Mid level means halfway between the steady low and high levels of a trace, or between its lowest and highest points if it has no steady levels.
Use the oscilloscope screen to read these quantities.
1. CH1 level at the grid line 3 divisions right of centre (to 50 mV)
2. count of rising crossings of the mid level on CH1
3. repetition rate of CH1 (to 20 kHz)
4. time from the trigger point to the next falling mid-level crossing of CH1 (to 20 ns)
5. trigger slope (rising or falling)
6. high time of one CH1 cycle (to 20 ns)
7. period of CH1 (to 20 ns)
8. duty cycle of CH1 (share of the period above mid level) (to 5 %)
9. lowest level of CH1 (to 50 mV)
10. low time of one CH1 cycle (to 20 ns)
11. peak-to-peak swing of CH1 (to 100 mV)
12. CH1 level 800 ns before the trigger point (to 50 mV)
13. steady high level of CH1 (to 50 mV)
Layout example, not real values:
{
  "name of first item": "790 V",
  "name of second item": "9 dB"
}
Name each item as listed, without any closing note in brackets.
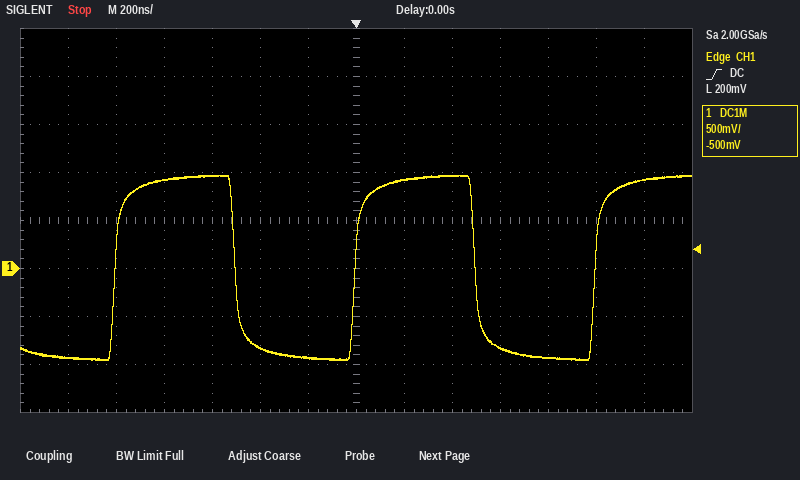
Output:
{
  "CH1 level at the grid line 3 divisions right of centre": "-850 mV",
  "count of rising crossings of the mid level on CH1": "3",
  "repetition rate of CH1": "1.00 MHz",
  "time from the trigger point to the next falling mid-level crossing of CH1": "500 ns",
  "trigger slope": "rising",
  "high time of one CH1 cycle": "500 ns",
  "period of CH1": "1.00 µs",
  "duty cycle of CH1 (share of the period above mid level)": "50 %",
  "lowest level of CH1": "-950 mV",
  "low time of one CH1 cycle": "500 ns",
  "peak-to-peak swing of CH1": "1.90 V",
  "CH1 level 800 ns before the trigger point": "900 mV",
  "steady high level of CH1": "950 mV"
}
